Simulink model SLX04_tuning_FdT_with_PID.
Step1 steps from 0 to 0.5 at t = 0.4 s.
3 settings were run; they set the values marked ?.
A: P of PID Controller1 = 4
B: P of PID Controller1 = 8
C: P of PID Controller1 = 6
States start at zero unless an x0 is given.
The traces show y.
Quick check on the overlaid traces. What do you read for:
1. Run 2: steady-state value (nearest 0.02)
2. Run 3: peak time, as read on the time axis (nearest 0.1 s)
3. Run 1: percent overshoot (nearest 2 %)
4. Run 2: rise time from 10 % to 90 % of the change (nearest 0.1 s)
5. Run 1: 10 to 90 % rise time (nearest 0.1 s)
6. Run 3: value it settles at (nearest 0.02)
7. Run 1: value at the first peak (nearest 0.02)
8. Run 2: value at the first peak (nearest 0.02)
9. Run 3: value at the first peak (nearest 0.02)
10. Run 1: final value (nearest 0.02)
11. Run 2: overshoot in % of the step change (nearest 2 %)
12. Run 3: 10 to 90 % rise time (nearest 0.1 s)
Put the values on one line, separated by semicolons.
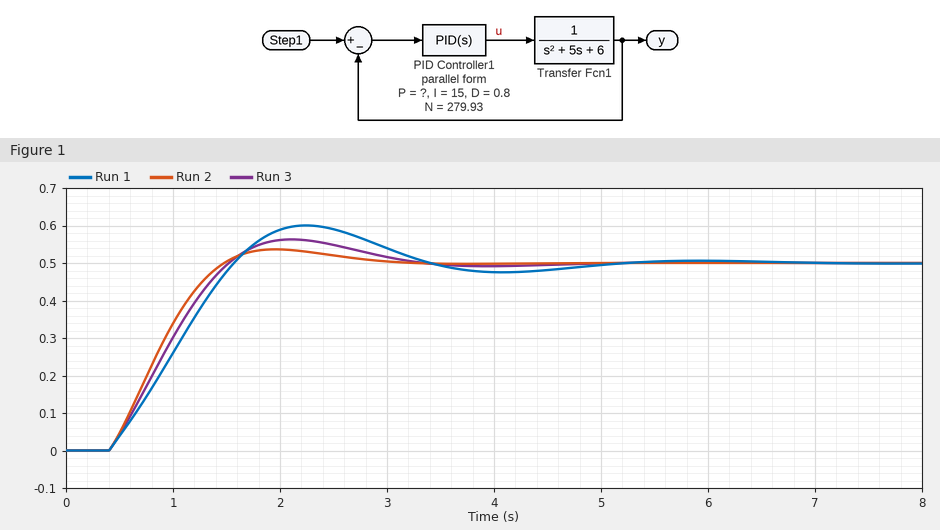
0.50; 2.1 s; 20 %; 0.8 s; 0.9 s; 0.50; 0.60; 0.54; 0.56; 0.50; 8 %; 0.8 s
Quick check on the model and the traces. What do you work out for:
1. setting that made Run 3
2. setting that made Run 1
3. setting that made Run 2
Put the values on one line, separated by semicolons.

C; A; B
